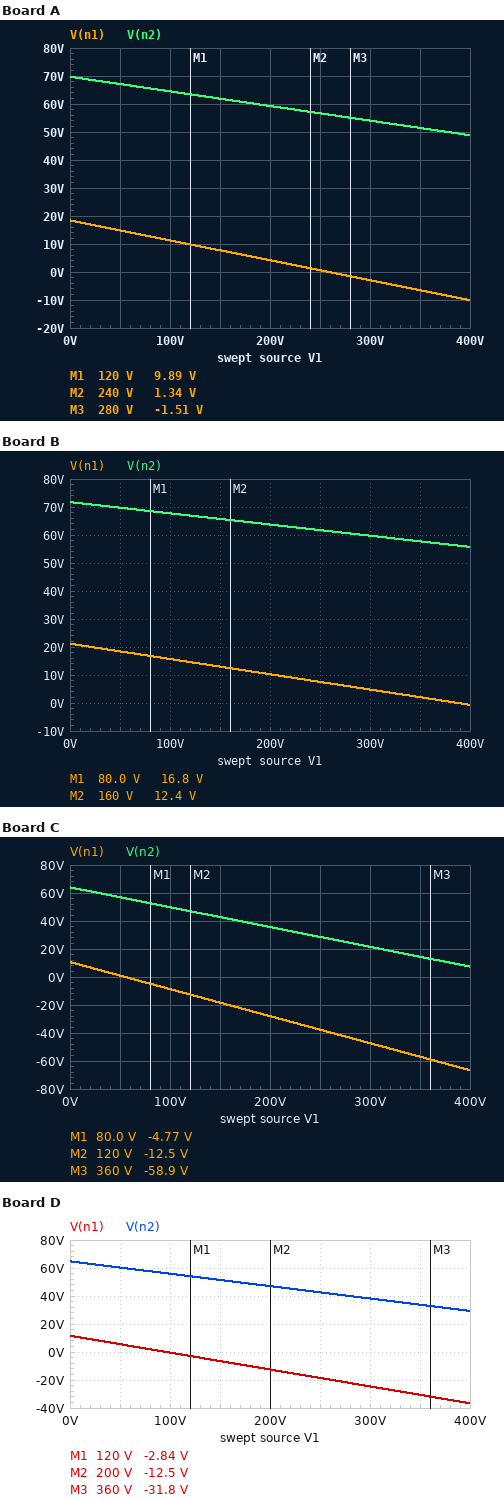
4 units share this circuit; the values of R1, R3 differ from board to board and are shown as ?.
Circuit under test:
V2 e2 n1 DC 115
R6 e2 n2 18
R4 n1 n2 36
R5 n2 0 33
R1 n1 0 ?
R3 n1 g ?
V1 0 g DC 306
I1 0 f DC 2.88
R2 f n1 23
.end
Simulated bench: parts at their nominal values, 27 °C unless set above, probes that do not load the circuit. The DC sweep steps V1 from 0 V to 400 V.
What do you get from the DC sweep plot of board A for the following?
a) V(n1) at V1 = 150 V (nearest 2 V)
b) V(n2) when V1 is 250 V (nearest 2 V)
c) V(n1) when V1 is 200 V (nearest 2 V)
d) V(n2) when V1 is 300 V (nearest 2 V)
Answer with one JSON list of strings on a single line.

["8 V", "56 V", "4 V", "54 V"]
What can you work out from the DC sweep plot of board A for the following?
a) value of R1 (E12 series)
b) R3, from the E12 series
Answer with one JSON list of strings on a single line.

["27 Ω", "220 Ω"]
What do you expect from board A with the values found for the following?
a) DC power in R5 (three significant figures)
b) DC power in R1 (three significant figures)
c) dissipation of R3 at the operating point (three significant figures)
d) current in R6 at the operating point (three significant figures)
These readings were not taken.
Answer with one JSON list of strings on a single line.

["87.6 W", "419 mW", "416 W", "3.22 A"]
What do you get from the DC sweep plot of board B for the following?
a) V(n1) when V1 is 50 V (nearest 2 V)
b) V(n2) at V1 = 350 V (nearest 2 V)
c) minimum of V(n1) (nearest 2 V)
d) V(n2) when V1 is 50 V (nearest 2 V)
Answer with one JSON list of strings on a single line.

["18 V", "58 V", "0 V", "70 V"]
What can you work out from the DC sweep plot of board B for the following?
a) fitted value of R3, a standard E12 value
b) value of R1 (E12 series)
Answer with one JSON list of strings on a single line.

["330 Ω", "33 Ω"]
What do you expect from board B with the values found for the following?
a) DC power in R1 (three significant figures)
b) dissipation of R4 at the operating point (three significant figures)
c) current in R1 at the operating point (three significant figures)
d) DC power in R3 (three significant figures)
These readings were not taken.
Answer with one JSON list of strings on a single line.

["609 mW", "84.1 W", "136 mA", "292 W"]
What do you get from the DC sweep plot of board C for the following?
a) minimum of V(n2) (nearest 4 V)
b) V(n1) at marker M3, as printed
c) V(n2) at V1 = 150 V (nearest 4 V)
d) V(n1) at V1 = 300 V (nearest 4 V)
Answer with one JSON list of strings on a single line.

["8 V", "-58.9 V", "44 V", "-48 V"]
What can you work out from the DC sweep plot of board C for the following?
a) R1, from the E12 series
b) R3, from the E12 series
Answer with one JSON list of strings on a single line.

["15 Ω", "47 Ω"]
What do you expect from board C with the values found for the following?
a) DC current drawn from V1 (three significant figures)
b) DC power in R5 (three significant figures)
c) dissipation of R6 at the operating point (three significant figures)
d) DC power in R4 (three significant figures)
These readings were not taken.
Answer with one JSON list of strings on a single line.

["5.48 A", "13.0 W", "117 W", "133 W"]
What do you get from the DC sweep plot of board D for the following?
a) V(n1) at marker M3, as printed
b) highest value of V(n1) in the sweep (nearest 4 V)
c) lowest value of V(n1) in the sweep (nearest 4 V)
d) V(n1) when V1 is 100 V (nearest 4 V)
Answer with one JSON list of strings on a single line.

["-31.8 V", "12 V", "-36 V", "0 V"]
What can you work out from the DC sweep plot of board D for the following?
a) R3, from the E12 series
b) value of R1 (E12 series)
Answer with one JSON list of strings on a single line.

["82 Ω", "15 Ω"]
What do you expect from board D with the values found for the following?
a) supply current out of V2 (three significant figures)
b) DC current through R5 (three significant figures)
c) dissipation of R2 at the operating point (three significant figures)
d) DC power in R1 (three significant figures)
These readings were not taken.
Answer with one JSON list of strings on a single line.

["2.89 A", "1.14 A", "191 W", "42.6 W"]
